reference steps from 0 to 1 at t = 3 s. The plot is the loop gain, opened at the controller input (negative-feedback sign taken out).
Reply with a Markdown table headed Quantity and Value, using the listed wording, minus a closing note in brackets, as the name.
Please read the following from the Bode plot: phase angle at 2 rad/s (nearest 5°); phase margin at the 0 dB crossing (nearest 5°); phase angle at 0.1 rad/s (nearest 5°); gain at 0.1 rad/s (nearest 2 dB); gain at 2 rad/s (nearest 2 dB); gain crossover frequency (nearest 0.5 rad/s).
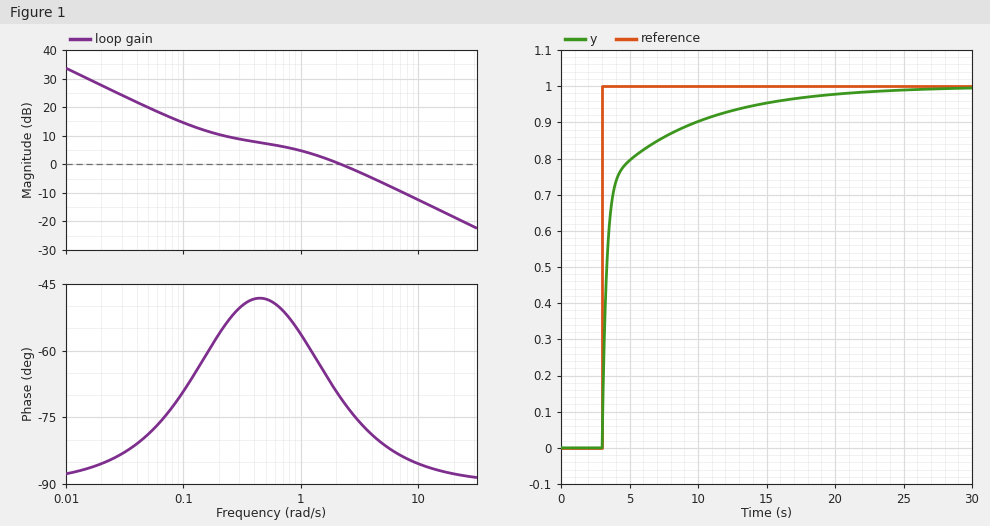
| Quantity | Value |
|---|---|
| phase angle at 2 rad/s | -70° |
| phase margin at the 0 dB crossing | 110° |
| phase angle at 0.1 rad/s | -70° |
| gain at 0.1 rad/s | 14 dB |
| gain at 2 rad/s | 0 dB |
| gain crossover frequency | 2.0 rad/s |
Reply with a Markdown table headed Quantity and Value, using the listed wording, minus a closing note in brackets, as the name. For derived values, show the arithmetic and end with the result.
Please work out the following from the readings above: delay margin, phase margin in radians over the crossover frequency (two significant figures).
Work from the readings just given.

| Quantity | Value |
|---|---|
| delay margin, phase margin in radians over the crossover frequency | 110 × π / 180 / 2 = 0.96 s |
